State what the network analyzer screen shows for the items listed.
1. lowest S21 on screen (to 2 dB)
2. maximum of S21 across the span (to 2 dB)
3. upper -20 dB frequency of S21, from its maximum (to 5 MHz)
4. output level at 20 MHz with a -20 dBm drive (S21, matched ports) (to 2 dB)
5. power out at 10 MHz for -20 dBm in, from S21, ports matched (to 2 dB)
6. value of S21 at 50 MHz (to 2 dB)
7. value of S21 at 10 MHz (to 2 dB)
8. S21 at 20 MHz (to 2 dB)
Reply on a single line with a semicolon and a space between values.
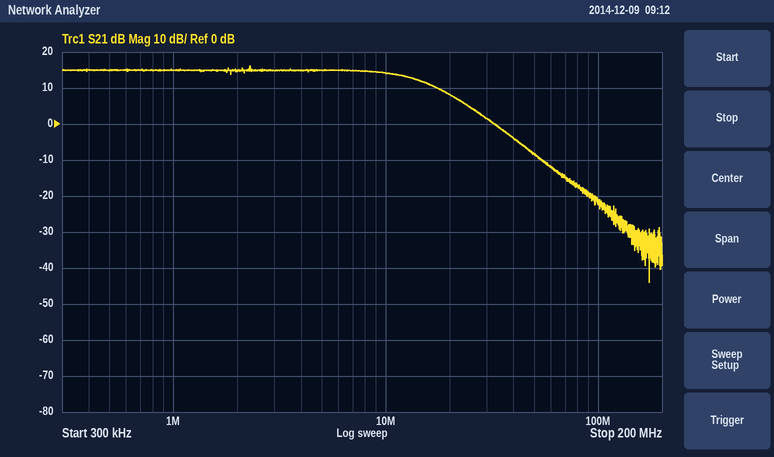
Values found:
-44 dB; 16 dB; 40 MHz; -12 dBm; -6 dBm; -8 dB; 14 dB; 8 dB
